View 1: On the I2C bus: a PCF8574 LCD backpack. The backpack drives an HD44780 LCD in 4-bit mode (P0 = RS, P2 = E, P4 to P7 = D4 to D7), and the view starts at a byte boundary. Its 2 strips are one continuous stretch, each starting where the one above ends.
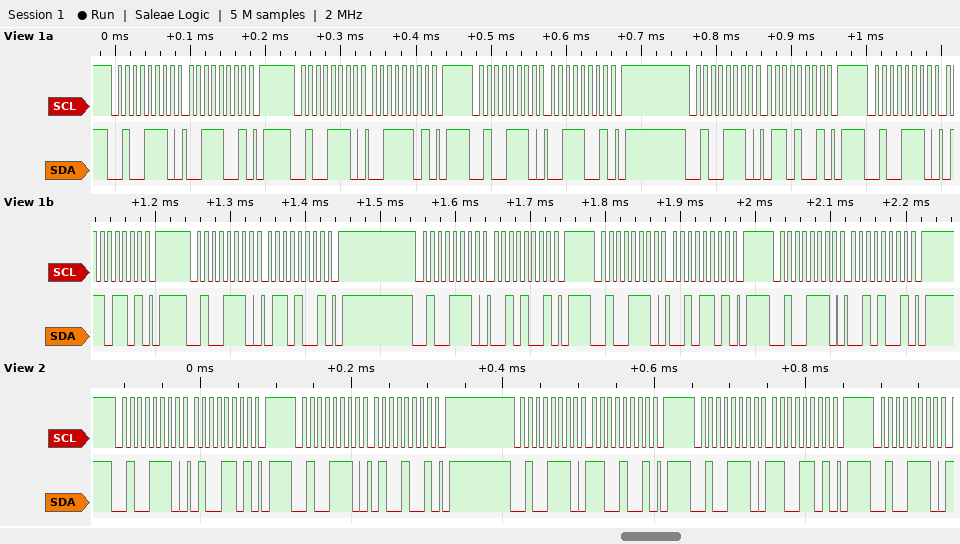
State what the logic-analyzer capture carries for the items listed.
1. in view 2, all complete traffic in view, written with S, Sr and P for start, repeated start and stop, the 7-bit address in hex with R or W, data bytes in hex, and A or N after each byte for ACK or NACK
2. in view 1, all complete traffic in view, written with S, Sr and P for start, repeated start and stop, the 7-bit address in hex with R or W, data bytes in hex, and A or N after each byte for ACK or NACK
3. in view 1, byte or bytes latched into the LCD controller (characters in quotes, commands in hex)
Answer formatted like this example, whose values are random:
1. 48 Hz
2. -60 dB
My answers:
1. S 27W A 4D A P S 27W A 49 A P S 27W A C9 A P S 27W A CD A P S 27W A
2. S 27W A 39 A P S 27W A 3D A P S 27W A 39 A P S 27W A 69 A P S 27W A 6D A P S 27W A 69 A P S 27W A 29 A P S 27W A 2D A P S 27W A 29 A P
3. '6'
